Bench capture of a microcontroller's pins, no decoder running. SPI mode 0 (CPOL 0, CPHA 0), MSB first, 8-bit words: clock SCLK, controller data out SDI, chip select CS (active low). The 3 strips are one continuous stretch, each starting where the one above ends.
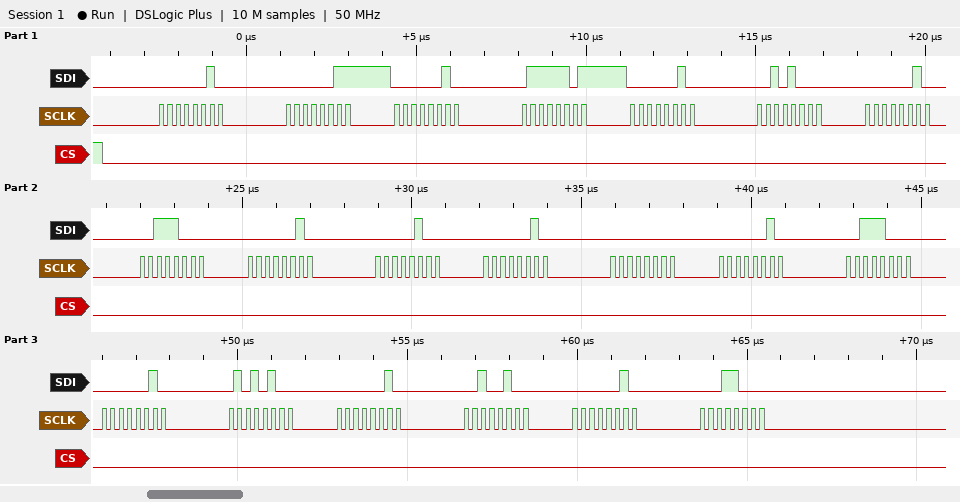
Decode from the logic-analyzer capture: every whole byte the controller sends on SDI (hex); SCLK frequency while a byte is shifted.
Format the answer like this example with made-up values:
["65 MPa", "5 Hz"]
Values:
["0x02 0x03 0x02 0x7D 0x02 0x28 0x02 0x38 0x02 0x04 0x02 0x00 0x02 0x38 0x02 0x54 0x02 0x24 0x02 0x18", "4 MHz"]
